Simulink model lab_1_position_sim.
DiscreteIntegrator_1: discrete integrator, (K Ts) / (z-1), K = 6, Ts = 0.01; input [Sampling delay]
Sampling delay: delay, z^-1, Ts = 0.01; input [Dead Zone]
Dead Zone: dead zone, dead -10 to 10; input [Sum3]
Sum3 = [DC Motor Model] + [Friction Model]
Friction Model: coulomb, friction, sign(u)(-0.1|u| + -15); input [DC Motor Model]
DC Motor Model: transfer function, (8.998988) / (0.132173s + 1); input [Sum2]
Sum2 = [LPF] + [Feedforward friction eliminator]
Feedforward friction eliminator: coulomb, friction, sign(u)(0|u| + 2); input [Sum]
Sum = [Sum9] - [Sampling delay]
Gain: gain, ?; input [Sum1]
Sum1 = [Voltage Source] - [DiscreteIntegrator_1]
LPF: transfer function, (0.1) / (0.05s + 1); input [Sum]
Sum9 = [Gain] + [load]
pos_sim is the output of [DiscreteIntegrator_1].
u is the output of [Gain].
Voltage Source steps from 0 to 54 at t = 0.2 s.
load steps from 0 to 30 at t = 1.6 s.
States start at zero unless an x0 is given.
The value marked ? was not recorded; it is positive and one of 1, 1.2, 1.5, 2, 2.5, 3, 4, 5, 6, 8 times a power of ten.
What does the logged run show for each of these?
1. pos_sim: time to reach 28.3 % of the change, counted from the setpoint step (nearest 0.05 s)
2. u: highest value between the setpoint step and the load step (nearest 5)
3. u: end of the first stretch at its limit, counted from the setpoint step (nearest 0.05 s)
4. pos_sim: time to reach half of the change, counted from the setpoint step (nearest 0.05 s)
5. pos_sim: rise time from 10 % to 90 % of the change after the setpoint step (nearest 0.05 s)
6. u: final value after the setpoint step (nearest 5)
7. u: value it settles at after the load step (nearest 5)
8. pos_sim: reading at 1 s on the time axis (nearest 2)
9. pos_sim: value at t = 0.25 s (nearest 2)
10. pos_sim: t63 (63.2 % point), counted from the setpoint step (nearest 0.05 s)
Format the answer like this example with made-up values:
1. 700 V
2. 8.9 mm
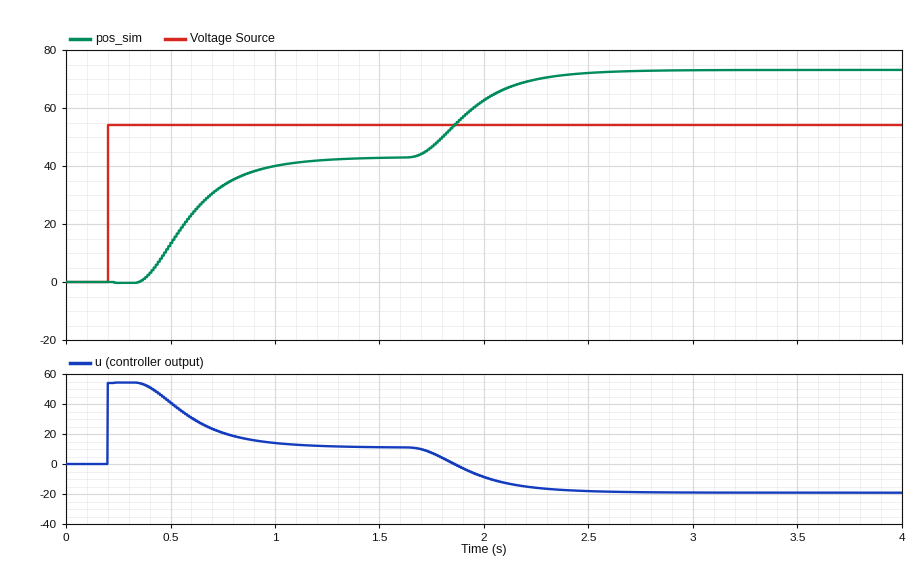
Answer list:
1. 0.30 s
2. 55
3. 0.15 s
4. 0.40 s
5. 0.50 s
6. 10
7. -20
8. 40
9. 0
10. 0.45 s
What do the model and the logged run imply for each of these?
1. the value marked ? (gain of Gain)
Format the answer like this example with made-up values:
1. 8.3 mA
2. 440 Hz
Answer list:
1. 1
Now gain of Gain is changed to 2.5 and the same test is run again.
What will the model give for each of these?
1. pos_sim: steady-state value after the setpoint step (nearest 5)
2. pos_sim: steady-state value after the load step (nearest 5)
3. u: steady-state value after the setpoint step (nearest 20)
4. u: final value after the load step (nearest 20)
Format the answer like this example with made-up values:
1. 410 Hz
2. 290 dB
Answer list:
1. 55
2. 65
3. 0
4. -20
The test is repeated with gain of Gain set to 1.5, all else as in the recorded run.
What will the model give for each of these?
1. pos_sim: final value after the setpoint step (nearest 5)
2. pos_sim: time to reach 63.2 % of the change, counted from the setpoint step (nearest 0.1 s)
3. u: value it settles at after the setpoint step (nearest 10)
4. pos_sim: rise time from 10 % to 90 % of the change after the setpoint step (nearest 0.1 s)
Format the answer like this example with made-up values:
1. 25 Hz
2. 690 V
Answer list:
1. 50
2. 0.3 s
3. 10
4. 0.3 s
